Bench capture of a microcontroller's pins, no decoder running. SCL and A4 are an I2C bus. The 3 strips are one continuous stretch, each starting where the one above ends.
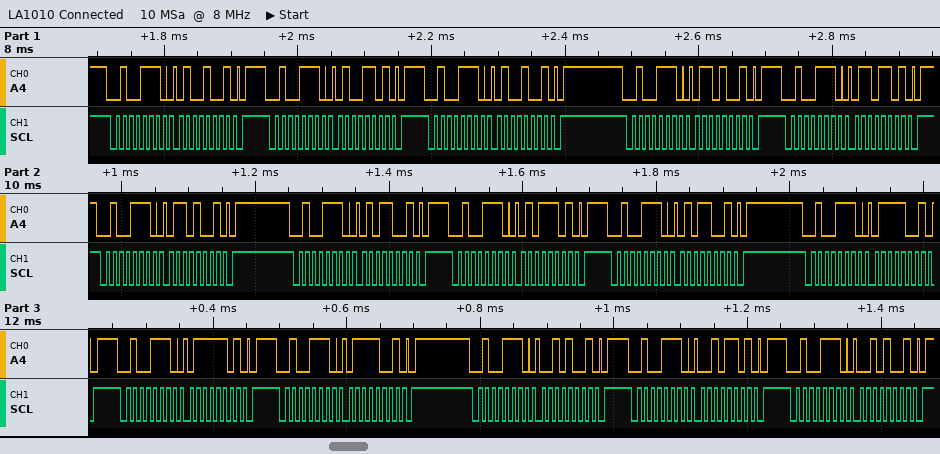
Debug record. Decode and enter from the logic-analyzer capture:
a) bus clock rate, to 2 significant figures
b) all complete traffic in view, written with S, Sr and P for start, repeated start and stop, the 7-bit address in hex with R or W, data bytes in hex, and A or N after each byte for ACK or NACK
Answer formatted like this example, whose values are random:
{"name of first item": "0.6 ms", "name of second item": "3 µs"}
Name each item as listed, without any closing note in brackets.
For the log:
{"bus clock rate, to 2 significant figures": "100 kHz", "all complete traffic in view, written with S, Sr and P for start, repeated start and stop, the 7-bit address in hex with R or W, data bytes in hex, and A or N after each byte for ACK or NACK": "S 27W A 49 A P S 27W A 4D A P S 27W A 49 A P S 27W A 69 A P S 27W A 6D A P S 27W A 69 A P S 27W A 59 A P S 27W A 5D A P S 27W A 59 A P S 27W A 79 A P S 27W A 7D A P S 27W A 79 A P S 27W A 29 A P S 27W A 2D A P S 27W A 29 A P"}
